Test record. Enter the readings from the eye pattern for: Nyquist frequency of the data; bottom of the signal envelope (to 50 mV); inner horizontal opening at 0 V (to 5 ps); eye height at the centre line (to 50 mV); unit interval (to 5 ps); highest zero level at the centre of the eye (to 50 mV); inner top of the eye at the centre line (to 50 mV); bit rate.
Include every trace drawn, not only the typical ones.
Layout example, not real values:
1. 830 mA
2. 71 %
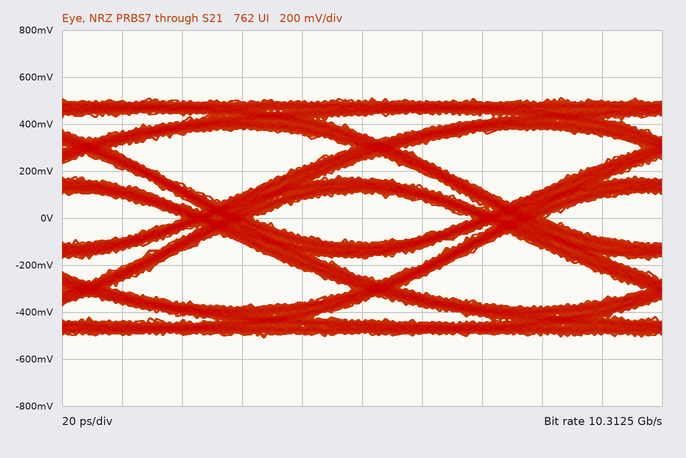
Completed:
1. 5.15625 GHz
2. -500 mV
3. 75 ps
4. 200 mV
5. 95 ps
6. -100 mV
7. 100 mV
8. 10.3125 Gb/s
